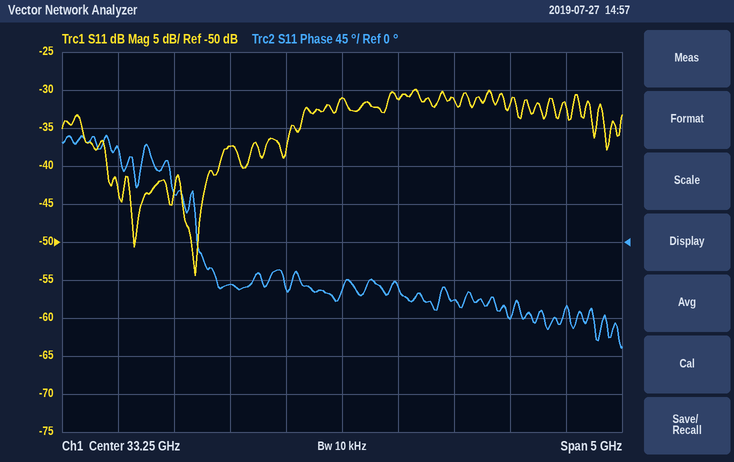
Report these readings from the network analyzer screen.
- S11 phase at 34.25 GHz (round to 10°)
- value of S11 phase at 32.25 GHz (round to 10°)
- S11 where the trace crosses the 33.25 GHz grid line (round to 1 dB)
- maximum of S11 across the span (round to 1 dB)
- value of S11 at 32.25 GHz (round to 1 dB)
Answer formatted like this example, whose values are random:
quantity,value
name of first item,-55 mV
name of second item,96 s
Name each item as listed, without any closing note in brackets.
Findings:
quantity,value
S11 phase at 34.25 GHz,-70°
value of S11 phase at 32.25 GHz,-50°
S11 where the trace crosses the 33.25 GHz grid line,-31 dB
maximum of S11 across the span,-30 dB
value of S11 at 32.25 GHz,-37 dB
